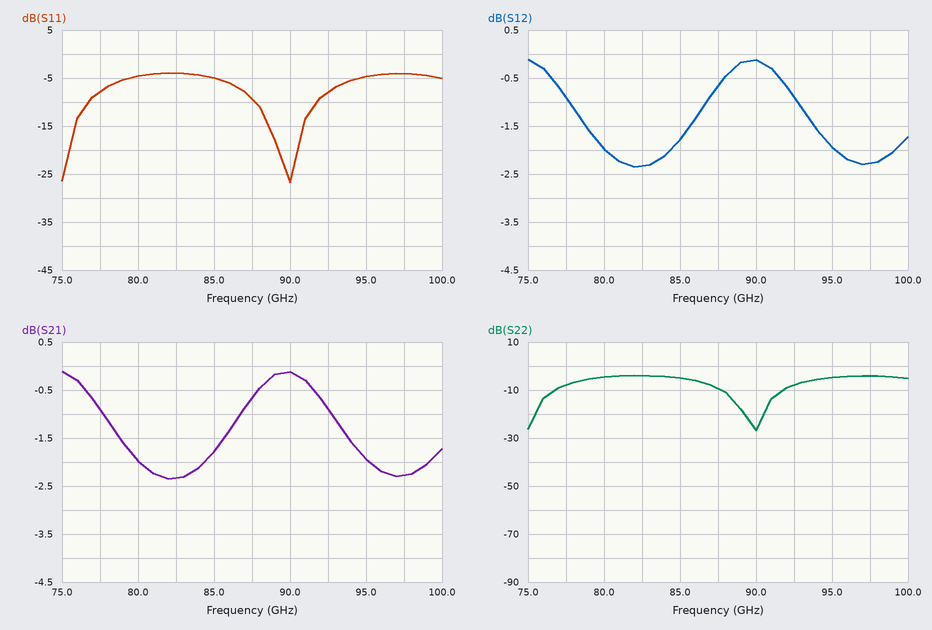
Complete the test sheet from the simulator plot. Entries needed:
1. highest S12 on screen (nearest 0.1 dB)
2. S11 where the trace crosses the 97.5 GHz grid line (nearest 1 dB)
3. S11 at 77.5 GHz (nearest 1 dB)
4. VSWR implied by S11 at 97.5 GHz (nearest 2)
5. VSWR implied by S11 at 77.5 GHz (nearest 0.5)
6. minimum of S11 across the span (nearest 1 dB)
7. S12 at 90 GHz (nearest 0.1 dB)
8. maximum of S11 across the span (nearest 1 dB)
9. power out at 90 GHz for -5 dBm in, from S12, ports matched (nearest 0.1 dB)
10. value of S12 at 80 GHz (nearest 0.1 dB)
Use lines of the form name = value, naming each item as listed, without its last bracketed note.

highest S12 on screen = -0.1 dB
S11 where the trace crosses the 97.5 GHz grid line = -4 dB
S11 at 77.5 GHz = -8 dB
VSWR implied by S11 at 97.5 GHz = 4
VSWR implied by S11 at 77.5 GHz = 2.5
minimum of S11 across the span = -27 dB
S12 at 90 GHz = -0.1 dB
maximum of S11 across the span = -4 dB
power out at 90 GHz for -5 dBm in, from S12, ports matched = -5.1 dBm
value of S12 at 80 GHz = -2.0 dB
